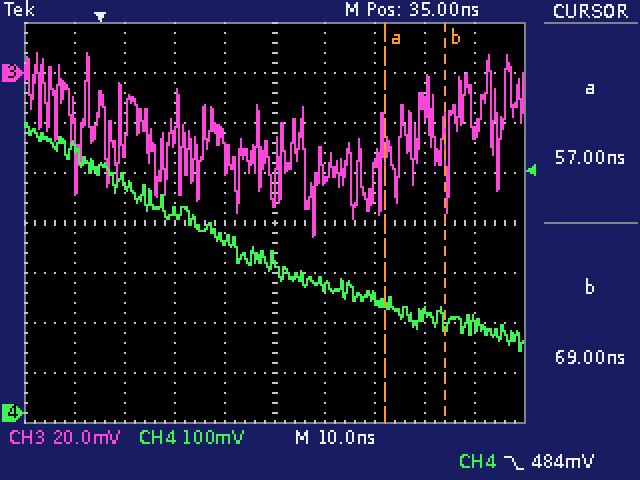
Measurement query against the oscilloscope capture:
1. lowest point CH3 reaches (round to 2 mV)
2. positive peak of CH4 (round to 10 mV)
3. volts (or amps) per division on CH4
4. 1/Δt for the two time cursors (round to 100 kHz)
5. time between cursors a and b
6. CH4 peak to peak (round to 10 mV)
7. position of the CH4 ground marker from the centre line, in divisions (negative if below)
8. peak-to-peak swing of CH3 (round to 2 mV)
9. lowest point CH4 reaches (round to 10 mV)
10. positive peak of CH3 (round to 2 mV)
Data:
-66 mV
580 mV
100 mV
83.3 MHz
12 ns
460 mV
-3.8 div
74 mV
120 mV
8 mV
